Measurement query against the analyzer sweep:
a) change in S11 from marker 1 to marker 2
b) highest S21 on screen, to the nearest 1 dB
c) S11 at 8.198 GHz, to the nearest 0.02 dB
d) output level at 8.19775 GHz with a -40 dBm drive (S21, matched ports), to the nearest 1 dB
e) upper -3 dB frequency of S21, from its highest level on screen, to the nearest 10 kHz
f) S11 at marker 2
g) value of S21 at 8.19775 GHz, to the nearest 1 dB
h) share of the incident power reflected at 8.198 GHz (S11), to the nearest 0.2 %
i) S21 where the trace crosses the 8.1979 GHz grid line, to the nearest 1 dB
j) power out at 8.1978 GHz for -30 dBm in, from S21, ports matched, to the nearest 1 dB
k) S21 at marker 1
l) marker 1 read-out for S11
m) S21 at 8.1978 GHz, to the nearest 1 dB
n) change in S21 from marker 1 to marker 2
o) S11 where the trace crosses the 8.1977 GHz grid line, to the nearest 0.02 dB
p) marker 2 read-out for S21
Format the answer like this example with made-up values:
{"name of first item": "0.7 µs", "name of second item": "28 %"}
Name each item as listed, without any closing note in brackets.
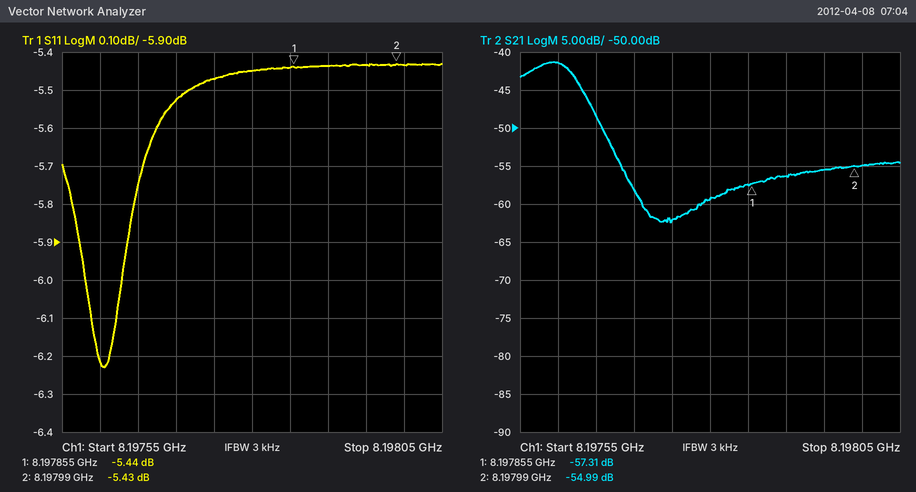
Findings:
{"change in S11 from marker 1 to marker 2": "0.01 dB", "highest S21 on screen, to the nearest 1 dB": "-41 dB", "S11 at 8.198 GHz, to the nearest 0.02 dB": "-5.44 dB", "output level at 8.19775 GHz with a -40 dBm drive (S21, matched ports), to the nearest 1 dB": "-102 dBm", "upper -3 dB frequency of S21, from its highest level on screen, to the nearest 10 kHz": "8.19763 GHz", "S11 at marker 2": "-5.43 dB", "value of S21 at 8.19775 GHz, to the nearest 1 dB": "-62 dB", "share of the incident power reflected at 8.198 GHz (S11), to the nearest 0.2 %": "28.6 %", "S21 where the trace crosses the 8.1979 GHz grid line, to the nearest 1 dB": "-56 dB", "power out at 8.1978 GHz for -30 dBm in, from S21, ports matched, to the nearest 1 dB": "-89 dBm", "S21 at marker 1": "-57.31 dB", "marker 1 read-out for S11": "-5.44 dB", "S21 at 8.1978 GHz, to the nearest 1 dB": "-59 dB", "change in S21 from marker 1 to marker 2": "2.32 dB", "S11 where the trace crosses the 8.1977 GHz grid line, to the nearest 0.02 dB": "-5.52 dB", "marker 2 read-out for S21": "-54.99 dB"}
